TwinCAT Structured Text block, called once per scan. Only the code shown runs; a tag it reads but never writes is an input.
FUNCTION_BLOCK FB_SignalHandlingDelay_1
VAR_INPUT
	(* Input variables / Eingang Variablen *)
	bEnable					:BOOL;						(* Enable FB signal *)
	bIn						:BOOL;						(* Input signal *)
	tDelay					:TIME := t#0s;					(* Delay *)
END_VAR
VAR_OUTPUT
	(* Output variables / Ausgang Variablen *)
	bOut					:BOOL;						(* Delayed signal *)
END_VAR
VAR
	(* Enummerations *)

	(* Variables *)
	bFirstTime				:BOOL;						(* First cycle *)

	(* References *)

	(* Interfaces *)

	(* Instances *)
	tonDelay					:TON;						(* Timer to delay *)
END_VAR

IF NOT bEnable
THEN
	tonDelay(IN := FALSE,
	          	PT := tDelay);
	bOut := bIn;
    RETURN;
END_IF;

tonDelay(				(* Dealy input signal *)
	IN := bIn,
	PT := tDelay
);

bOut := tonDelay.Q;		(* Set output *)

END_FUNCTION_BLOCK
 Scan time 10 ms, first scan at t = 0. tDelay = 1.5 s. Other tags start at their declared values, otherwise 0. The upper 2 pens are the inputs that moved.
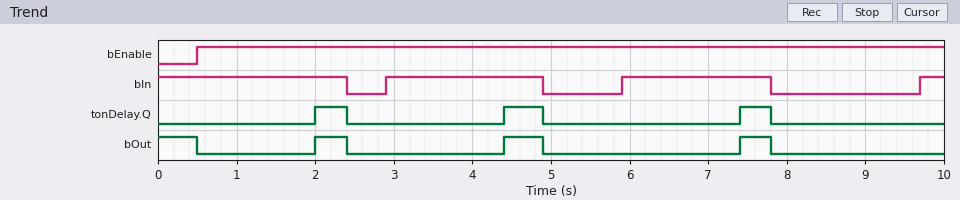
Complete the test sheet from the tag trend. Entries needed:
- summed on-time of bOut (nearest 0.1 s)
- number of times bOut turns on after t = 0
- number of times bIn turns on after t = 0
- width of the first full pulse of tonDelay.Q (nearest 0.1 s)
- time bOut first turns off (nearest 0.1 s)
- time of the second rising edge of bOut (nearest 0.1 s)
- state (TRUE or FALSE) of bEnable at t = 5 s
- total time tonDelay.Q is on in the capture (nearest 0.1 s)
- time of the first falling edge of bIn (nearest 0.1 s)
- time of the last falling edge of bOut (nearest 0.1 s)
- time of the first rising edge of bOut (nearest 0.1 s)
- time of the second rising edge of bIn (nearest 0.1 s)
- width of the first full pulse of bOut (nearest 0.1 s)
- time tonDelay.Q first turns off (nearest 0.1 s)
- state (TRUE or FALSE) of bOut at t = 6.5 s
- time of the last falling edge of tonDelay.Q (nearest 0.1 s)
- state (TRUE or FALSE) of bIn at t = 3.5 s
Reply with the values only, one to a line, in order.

1.8 s
3
3
0.4 s
0.5 s
4.4 s
TRUE
1.3 s
2.4 s
7.8 s
2.0 s
5.9 s
0.4 s
2.4 s
FALSE
7.8 s
TRUE
